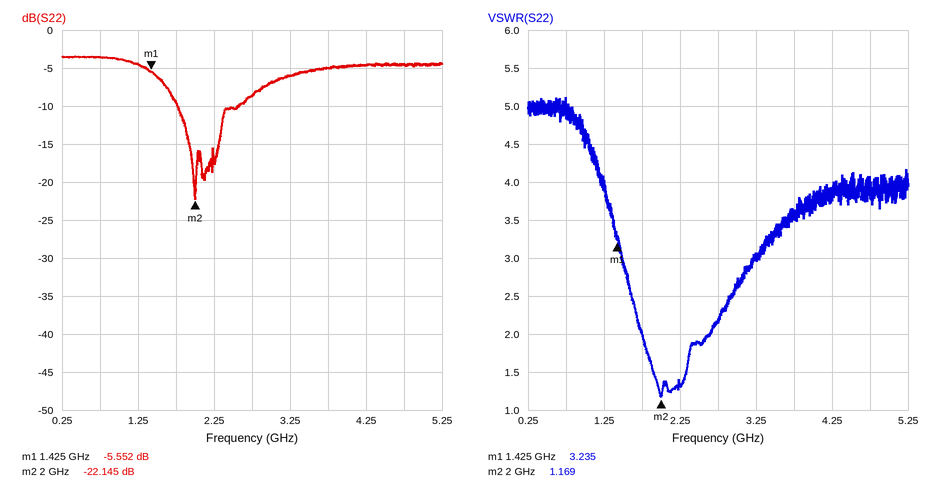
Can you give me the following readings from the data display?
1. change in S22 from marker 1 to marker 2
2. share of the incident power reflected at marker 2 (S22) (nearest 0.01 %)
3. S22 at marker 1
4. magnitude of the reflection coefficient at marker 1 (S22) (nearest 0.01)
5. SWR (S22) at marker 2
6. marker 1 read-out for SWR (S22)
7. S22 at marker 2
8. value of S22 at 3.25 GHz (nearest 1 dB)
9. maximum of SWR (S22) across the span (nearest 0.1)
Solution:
-16.593 dB
0.61 %
-5.552 dB
0.53
1.169
3.235
-22.145 dB
-6 dB
5.1
